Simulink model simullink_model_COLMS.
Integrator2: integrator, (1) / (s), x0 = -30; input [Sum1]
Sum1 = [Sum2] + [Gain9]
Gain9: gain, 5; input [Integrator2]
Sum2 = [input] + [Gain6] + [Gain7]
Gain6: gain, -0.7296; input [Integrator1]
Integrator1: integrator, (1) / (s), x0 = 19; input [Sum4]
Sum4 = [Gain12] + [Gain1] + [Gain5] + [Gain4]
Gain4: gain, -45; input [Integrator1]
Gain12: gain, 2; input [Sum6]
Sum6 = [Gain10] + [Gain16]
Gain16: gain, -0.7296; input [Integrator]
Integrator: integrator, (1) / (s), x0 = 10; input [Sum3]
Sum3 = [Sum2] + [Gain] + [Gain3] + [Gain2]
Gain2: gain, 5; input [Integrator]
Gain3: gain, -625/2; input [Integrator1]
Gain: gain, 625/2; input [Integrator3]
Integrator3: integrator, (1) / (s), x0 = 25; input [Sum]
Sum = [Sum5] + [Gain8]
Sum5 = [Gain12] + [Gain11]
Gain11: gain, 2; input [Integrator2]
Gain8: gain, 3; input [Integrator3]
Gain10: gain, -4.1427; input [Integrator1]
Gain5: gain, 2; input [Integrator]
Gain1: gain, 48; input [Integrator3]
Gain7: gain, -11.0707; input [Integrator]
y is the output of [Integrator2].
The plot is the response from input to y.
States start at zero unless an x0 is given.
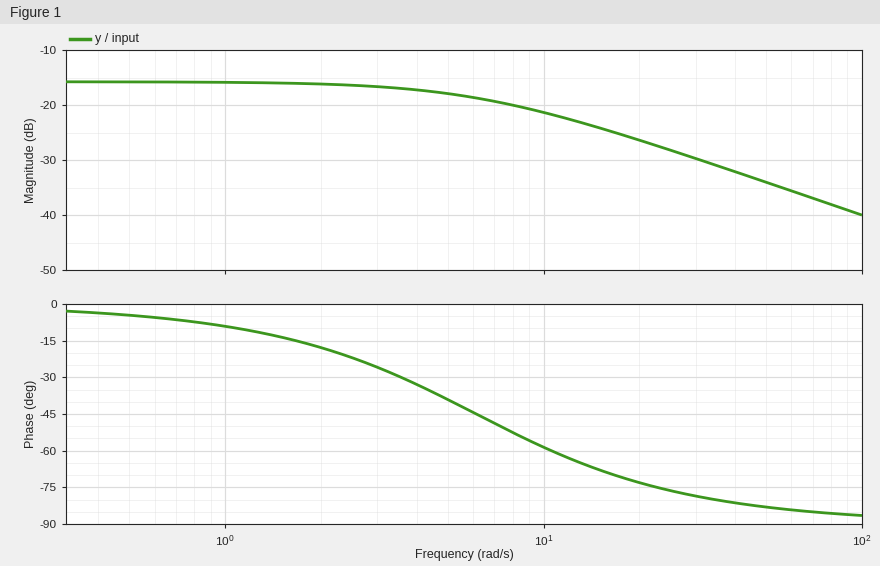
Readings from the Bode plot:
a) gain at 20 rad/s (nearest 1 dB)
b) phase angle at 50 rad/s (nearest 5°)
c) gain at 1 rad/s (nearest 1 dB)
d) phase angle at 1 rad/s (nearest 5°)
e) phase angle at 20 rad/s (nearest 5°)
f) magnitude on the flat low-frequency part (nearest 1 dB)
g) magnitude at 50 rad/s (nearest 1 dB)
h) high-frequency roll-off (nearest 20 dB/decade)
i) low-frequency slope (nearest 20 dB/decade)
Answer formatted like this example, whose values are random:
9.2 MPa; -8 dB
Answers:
-26 dB; -85°; -16 dB; -10°; -75°; -16 dB; -34 dB; -20 dB/decade; 0 dB/decade
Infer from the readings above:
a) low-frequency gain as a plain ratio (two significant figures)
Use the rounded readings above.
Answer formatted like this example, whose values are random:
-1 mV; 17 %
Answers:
0.16
